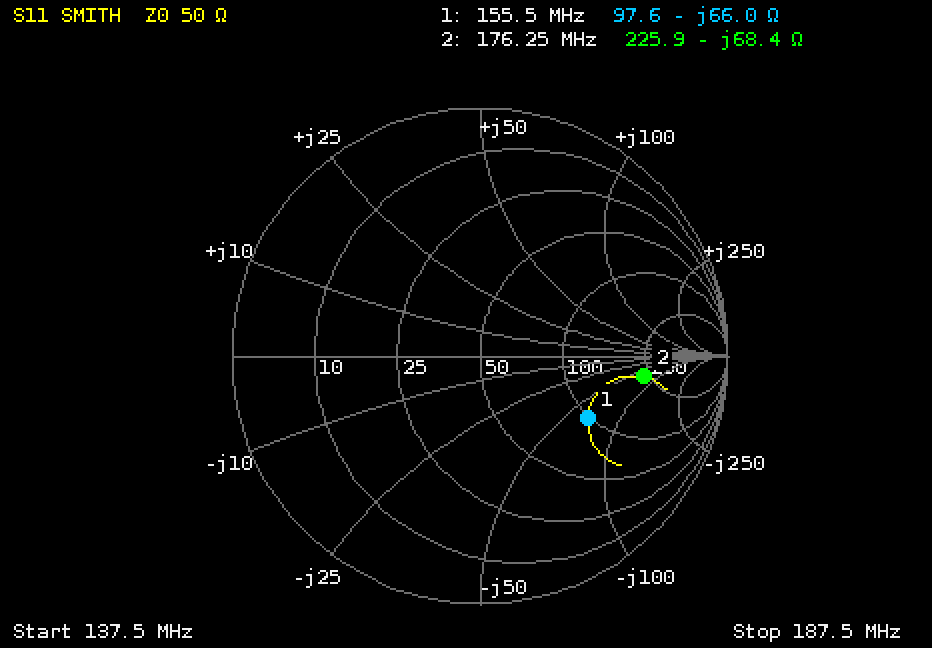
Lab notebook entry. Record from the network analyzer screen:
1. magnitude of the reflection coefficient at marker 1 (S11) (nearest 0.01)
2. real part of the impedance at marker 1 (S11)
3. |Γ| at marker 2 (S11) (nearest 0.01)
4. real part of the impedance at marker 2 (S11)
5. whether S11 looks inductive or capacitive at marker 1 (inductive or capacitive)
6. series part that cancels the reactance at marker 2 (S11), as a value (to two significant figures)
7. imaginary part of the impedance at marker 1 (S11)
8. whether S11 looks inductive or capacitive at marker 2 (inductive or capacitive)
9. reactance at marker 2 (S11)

0.50
97.6 Ω
0.66
225.9 Ω
capacitive
62 nH
-66.0 Ω
capacitive
-68.4 Ω
